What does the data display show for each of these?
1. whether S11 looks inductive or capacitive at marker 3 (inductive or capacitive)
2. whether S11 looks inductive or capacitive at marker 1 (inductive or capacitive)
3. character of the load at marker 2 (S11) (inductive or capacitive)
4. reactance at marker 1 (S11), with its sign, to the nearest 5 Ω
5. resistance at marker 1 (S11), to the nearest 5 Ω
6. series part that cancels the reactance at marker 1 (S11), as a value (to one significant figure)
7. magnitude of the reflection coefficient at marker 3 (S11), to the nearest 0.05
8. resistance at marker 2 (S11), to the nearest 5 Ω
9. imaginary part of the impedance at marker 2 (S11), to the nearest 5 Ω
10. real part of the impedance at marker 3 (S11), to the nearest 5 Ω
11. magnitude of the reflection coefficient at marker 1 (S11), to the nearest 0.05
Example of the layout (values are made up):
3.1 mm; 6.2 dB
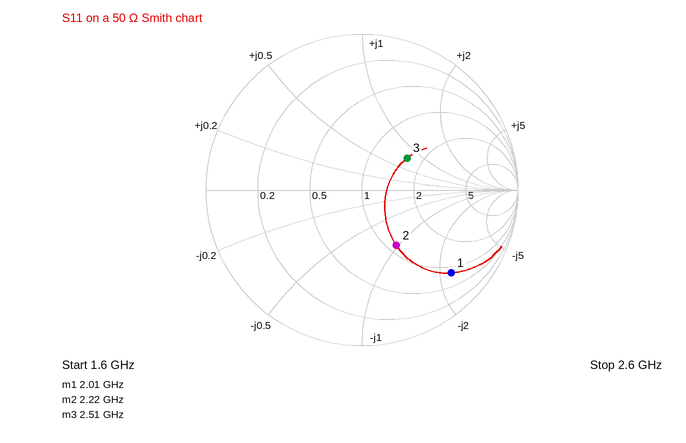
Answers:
inductive; capacitive; capacitive; -115 Ω; 40 Ω; 9 nH; 0.35; 55 Ω; -50 Ω; 80 Ω; 0.80
